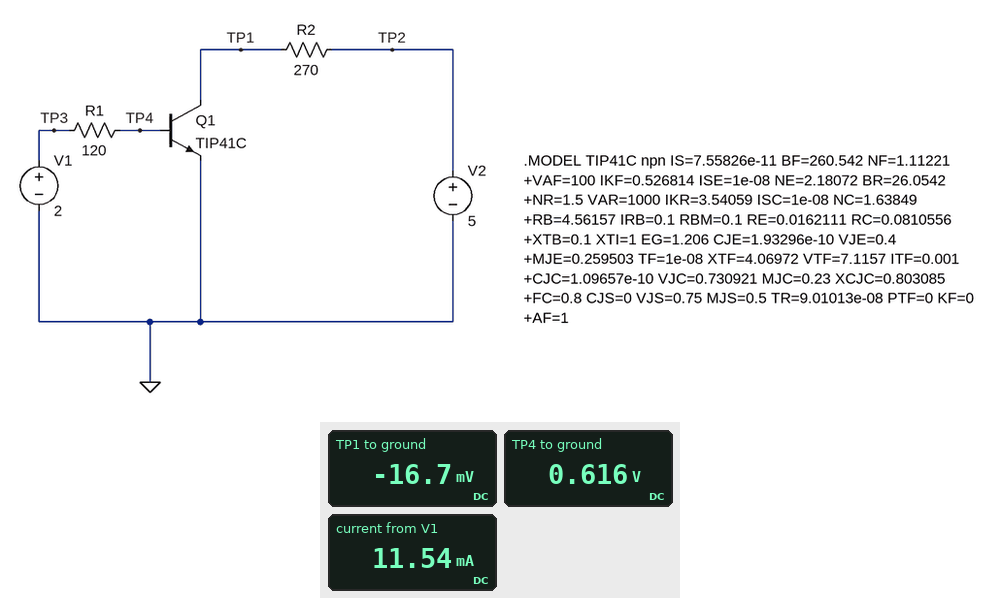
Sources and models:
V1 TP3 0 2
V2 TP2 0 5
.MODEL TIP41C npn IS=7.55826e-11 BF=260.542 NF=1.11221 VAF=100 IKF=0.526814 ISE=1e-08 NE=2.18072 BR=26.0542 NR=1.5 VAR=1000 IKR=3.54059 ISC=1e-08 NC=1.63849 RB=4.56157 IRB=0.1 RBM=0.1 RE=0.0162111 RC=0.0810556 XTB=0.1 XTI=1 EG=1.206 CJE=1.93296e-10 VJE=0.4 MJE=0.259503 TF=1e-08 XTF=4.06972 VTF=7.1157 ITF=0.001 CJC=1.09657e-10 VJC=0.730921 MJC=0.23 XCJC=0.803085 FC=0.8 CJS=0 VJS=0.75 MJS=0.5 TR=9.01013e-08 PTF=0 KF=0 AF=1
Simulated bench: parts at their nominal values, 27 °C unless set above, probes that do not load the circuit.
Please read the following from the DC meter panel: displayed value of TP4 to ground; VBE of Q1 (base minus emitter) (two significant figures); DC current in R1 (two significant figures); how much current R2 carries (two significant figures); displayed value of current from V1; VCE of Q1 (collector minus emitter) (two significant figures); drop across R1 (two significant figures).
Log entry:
0.616 V
620 mV
12 mA
19 mA
11.54 mA
-17 mV
1.4 V
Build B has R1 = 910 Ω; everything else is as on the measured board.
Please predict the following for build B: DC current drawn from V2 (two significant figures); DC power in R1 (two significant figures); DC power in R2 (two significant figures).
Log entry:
18 mA
2.3 mW
90 mW
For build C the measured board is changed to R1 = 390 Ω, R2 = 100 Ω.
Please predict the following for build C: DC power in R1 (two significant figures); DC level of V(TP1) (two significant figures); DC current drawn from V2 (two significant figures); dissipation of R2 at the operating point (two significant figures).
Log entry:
5.0 mW
59 mV
49 mA
240 mW
